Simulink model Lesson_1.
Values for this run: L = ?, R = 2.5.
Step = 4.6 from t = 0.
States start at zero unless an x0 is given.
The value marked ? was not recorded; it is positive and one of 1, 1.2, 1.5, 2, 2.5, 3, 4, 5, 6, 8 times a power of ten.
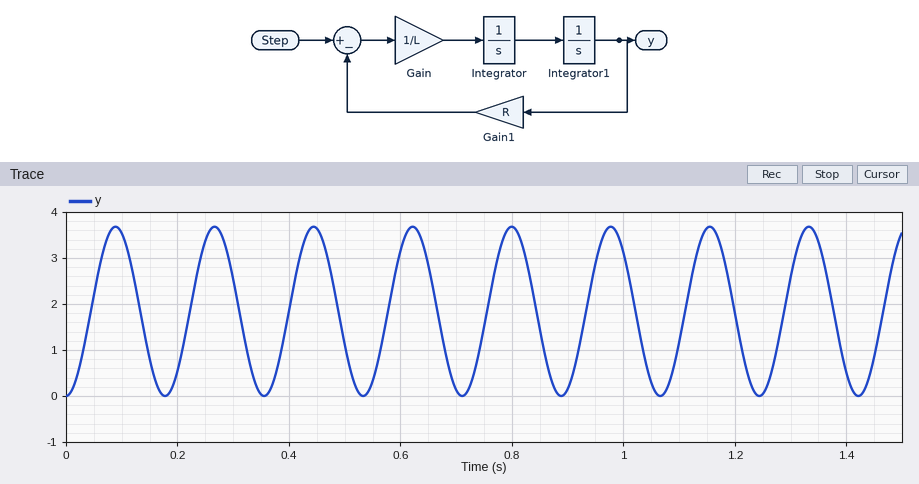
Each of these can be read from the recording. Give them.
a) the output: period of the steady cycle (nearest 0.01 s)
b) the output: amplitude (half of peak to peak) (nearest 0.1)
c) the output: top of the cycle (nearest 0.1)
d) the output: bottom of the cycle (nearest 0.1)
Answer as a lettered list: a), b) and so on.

a) 0.18 s
b) 1.8
c) 3.7
d) 0.0
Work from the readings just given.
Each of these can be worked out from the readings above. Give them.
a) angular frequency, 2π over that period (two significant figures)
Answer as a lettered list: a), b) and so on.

a) 35 rad/s
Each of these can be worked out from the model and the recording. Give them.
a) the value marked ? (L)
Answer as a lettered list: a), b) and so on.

a) 0.002
